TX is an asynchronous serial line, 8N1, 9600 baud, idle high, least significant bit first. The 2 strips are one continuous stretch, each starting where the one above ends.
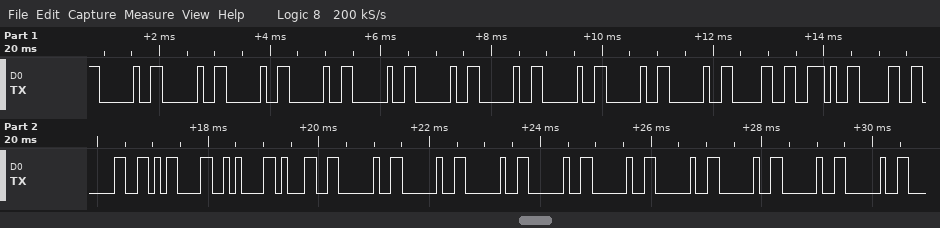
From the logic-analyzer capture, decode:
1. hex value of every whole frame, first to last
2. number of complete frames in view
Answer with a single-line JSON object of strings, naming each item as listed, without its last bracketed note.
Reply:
{"hex value of every whole frame, first to last": "20 20 20 20 20 20 20 20 20 20 30 2E 30 30 0D 0A 31 20 20 20 20 20 20 20 20 20", "number of complete frames in view": "26"}
